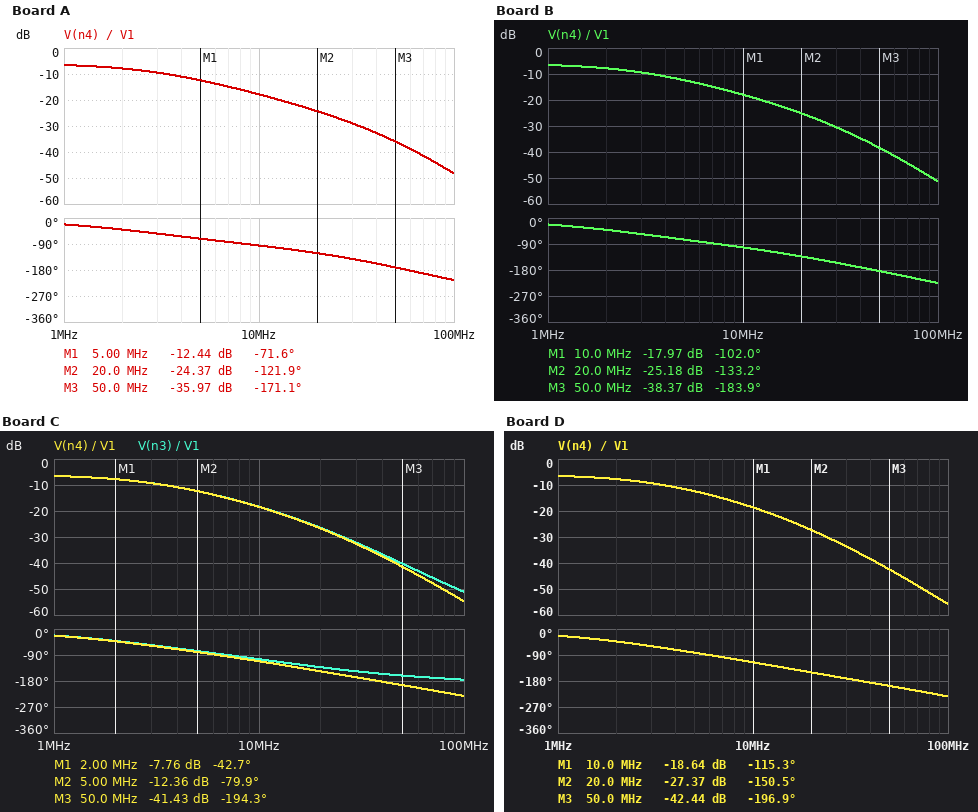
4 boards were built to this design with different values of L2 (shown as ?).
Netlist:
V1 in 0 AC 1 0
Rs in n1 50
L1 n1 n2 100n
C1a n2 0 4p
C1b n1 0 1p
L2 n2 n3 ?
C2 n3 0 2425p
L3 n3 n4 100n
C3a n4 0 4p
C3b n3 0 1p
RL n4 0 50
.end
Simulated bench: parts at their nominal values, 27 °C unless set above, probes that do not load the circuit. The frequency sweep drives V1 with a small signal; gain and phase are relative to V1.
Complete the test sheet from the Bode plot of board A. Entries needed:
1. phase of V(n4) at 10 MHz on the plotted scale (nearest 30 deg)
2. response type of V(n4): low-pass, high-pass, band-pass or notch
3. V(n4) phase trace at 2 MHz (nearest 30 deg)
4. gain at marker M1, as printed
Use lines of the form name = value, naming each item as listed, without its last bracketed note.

phase of V(n4) at 10 MHz on the plotted scale = -90 deg
response type of V(n4): low-pass, high-pass, band-pass or notch = low-pass
V(n4) phase trace at 2 MHz = -30 deg
gain at marker M1, as printed = -12.44 dB
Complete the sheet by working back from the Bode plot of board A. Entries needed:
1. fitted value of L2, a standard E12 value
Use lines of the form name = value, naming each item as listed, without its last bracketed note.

fitted value of L2, a standard E12 value = 82 nH
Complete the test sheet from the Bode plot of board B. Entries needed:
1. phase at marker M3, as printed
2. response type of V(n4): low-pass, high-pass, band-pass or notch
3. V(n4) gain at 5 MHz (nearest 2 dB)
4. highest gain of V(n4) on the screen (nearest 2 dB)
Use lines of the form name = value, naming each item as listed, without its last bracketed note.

phase at marker M3, as printed = -183.9 deg
response type of V(n4): low-pass, high-pass, band-pass or notch = low-pass
V(n4) gain at 5 MHz = -12 dB
highest gain of V(n4) on the screen = -6 dB
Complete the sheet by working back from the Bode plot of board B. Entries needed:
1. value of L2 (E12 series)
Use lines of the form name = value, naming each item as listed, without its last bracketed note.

value of L2 = 180 nH
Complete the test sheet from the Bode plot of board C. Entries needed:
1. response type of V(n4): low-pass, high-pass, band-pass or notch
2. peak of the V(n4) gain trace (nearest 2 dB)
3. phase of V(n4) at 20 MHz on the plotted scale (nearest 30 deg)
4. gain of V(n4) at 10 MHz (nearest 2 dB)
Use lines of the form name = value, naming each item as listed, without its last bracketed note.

response type of V(n4): low-pass, high-pass, band-pass or notch = low-pass
peak of the V(n4) gain trace = -6 dB
phase of V(n4) at 20 MHz on the plotted scale = -150 deg
gain of V(n4) at 10 MHz = -18 dB
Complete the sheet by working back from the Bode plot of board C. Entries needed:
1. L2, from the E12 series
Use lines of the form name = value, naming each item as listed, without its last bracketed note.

L2, from the E12 series = 330 nH
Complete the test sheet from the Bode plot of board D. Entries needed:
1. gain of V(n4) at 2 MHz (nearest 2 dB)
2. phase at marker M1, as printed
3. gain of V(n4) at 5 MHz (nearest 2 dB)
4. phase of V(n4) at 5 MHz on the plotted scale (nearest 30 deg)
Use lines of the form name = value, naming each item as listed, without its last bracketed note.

gain of V(n4) at 2 MHz = -8 dB
phase at marker M1, as printed = -115.3 deg
gain of V(n4) at 5 MHz = -12 dB
phase of V(n4) at 5 MHz on the plotted scale = -90 deg
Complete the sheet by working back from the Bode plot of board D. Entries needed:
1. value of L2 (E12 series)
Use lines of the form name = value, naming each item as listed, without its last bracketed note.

value of L2 = 390 nH
